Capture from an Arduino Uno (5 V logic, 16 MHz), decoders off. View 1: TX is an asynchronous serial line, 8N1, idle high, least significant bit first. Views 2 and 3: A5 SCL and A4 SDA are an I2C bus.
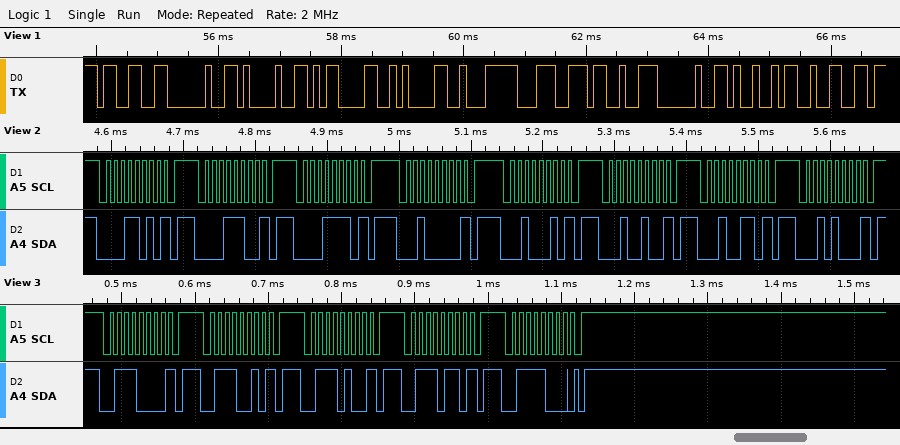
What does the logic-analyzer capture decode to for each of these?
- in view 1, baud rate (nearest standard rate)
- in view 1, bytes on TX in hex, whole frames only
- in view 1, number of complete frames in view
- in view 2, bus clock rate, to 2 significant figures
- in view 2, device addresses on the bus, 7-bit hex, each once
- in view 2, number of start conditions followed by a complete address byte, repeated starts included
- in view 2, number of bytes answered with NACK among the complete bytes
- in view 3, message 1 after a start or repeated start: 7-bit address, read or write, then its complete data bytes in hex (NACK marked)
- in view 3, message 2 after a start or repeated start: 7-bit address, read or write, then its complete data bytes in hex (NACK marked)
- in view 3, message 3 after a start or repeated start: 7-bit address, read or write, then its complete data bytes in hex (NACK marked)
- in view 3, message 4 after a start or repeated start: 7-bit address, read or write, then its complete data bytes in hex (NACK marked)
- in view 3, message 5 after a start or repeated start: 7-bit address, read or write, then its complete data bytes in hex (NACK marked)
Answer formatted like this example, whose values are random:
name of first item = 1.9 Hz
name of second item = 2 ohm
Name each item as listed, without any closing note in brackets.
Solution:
in view 1, baud rate = 9600 baud
in view 1, bytes on TX in hex, whole frames only = 33 20 21 0D 0A E2 9C 93 20 49 32
in view 1, number of complete frames in view = 11
in view 2, bus clock rate, to 2 significant figures = 100 kHz
in view 2, device addresses on the bus, 7-bit hex, each once = 0x0D 0x0E 0x0F 0x10 0x11 0x12 0x13 0x14
in view 2, number of start conditions followed by a complete address byte, repeated starts included = 8
in view 2, number of bytes answered with NACK among the complete bytes = 8
in view 3, message 1 after a start or repeated start: 7-bit address, read or write, then its complete data bytes in hex = 0x38 write NACK
in view 3, message 2 after a start or repeated start: 7-bit address, read or write, then its complete data bytes in hex = 0x39 write NACK
in view 3, message 3 after a start or repeated start: 7-bit address, read or write, then its complete data bytes in hex = 0x3A write NACK
in view 3, message 4 after a start or repeated start: 7-bit address, read or write, then its complete data bytes in hex = 0x3B write NACK
in view 3, message 5 after a start or repeated start: 7-bit address, read or write, then its complete data bytes in hex = 0x3C write
